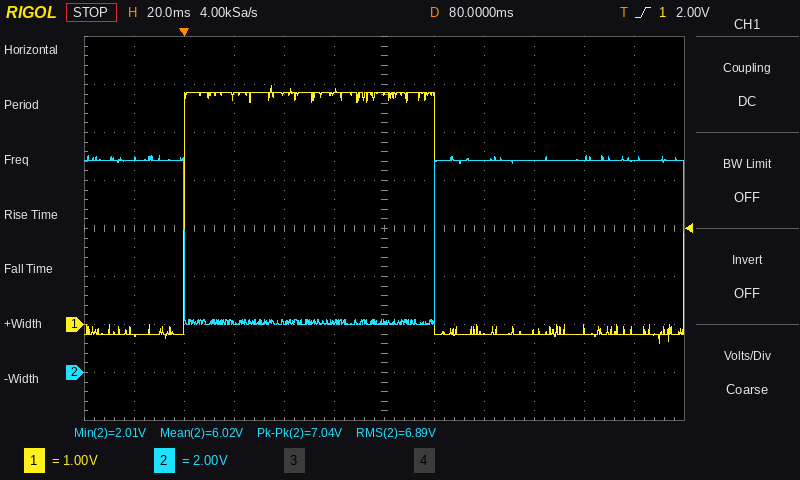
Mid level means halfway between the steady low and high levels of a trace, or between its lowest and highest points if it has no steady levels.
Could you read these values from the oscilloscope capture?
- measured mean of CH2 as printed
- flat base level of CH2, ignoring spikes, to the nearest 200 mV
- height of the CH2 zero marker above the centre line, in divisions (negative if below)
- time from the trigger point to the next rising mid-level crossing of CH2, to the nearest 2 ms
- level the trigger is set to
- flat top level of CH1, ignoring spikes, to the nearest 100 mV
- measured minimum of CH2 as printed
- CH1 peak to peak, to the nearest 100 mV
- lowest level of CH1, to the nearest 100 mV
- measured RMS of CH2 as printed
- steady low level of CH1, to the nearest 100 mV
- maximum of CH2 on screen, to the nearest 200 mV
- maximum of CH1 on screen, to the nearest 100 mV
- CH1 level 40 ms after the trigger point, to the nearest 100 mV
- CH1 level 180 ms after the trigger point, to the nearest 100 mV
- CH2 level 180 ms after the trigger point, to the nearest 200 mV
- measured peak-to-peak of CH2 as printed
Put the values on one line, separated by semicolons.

6.02 V; 2.0 V; -3.0 div; 100 ms; 2.00 V; 4.8 V; 2.01 V; 5.4 V; -400 mV; 6.89 V; -200 mV; 9.0 V; 5.0 V; 4.8 V; -100 mV; 8.8 V; 7.04 V
